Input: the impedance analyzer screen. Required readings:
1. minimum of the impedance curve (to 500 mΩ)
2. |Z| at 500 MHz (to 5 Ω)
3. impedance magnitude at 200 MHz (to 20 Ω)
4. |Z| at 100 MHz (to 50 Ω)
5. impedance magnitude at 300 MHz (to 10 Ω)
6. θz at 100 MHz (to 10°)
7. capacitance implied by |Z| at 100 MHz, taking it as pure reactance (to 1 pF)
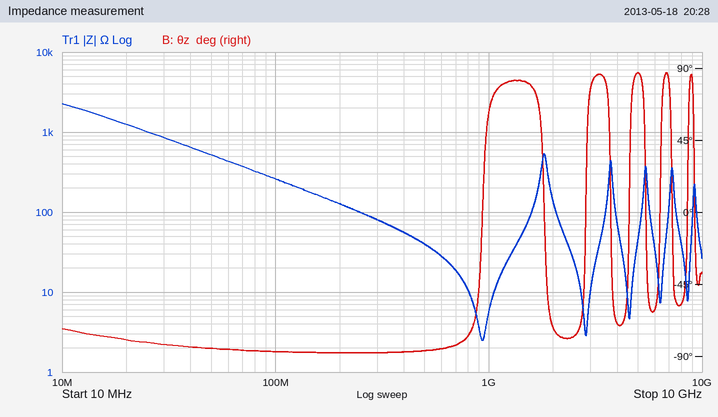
2.5 Ω
40 Ω
120 Ω
250 Ω
80 Ω
-90°
6 pF
